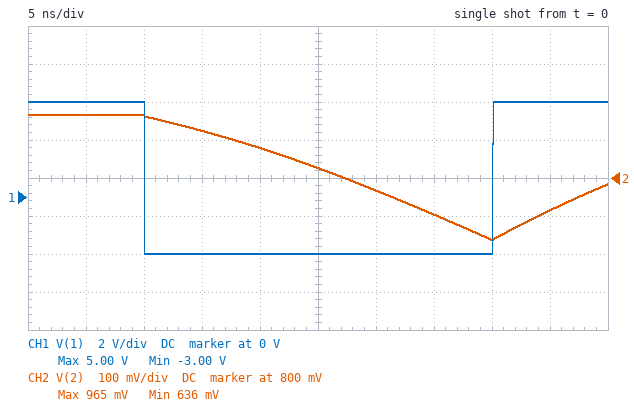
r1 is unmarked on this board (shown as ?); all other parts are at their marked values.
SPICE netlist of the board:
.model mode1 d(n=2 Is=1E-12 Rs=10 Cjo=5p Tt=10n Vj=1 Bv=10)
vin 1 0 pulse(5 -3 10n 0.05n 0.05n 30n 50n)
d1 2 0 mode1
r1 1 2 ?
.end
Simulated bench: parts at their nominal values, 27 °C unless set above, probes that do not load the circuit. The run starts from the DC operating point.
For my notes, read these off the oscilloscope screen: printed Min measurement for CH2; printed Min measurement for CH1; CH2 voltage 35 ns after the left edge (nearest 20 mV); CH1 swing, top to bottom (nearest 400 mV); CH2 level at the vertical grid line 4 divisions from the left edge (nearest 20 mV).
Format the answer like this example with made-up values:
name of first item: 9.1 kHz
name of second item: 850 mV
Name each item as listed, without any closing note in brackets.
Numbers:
printed Min measurement for CH2: 636 mV
printed Min measurement for CH1: -3.00 V
CH2 voltage 35 ns after the left edge: 700 mV
CH1 swing, top to bottom: 8.0 V
CH2 level at the vertical grid line 4 divisions from the left edge: 880 mV
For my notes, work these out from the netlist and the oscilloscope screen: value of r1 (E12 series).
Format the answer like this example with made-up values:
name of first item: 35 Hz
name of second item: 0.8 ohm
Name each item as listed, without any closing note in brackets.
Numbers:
value of r1: 33 kΩ
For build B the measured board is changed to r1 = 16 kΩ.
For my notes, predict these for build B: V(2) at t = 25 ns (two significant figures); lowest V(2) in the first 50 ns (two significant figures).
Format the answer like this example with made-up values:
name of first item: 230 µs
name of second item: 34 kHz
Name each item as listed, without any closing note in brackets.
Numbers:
V(2) at t = 25 ns: 760 mV
lowest V(2) in the first 50 ns: 310 mV
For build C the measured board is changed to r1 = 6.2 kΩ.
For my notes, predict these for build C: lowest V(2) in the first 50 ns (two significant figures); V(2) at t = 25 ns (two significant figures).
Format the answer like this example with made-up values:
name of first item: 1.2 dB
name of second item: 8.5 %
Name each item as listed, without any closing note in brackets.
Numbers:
lowest V(2) in the first 50 ns: -980 mV
V(2) at t = 25 ns: 450 mV
